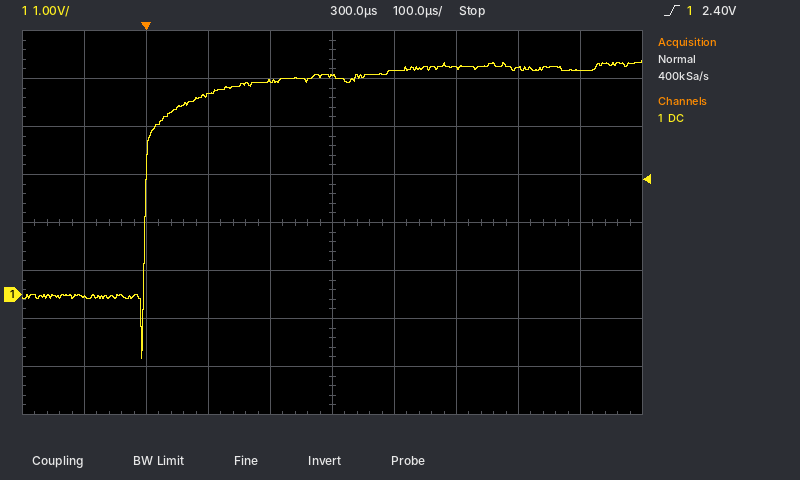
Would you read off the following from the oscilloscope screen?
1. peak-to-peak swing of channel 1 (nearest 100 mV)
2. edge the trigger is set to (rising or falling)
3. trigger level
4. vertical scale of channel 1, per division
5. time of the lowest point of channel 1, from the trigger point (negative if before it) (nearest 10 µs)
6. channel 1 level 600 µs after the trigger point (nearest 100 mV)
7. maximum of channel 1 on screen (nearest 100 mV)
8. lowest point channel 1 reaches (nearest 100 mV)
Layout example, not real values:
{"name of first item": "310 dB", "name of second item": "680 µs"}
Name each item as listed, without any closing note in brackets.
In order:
{"peak-to-peak swing of channel 1": "6.2 V", "edge the trigger is set to": "rising", "trigger level": "2.40 V", "vertical scale of channel 1, per division": "1 V", "time of the lowest point of channel 1, from the trigger point (negative if before it)": "-10 µs", "channel 1 level 600 µs after the trigger point": "4.7 V", "maximum of channel 1 on screen": "4.9 V", "lowest point channel 1 reaches": "-1.3 V"}
